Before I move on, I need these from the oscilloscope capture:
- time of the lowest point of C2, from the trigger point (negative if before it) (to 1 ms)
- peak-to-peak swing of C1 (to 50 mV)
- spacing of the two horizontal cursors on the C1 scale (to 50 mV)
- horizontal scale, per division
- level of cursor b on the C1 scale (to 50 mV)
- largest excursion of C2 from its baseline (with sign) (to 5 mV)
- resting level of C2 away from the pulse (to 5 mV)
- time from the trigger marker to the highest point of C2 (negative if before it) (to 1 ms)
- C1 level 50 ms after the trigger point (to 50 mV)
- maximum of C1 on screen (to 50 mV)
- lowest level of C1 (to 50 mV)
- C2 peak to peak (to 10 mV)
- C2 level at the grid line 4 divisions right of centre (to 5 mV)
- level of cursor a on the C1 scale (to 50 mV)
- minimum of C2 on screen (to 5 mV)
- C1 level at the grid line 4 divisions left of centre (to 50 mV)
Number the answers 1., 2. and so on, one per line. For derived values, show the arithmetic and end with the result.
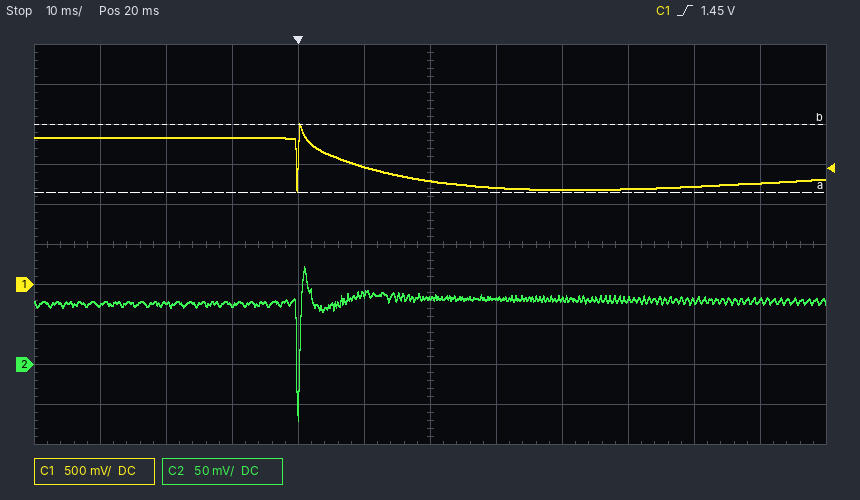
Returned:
1. 0 ms
2. 2.00 V − (1.15 V) = 850 mV
3. 850 mV
4. 10 ms
5. 2.00 V
6. -70 mV − (80 mV) = -150 mV
7. 80 mV
8. +1 ms
9. 1.20 V
10. 2.00 V
11. 1.15 V
12. 190 mV
13. 80 mV
14. 1.15 V
15. -70 mV
16. 1.85 V
